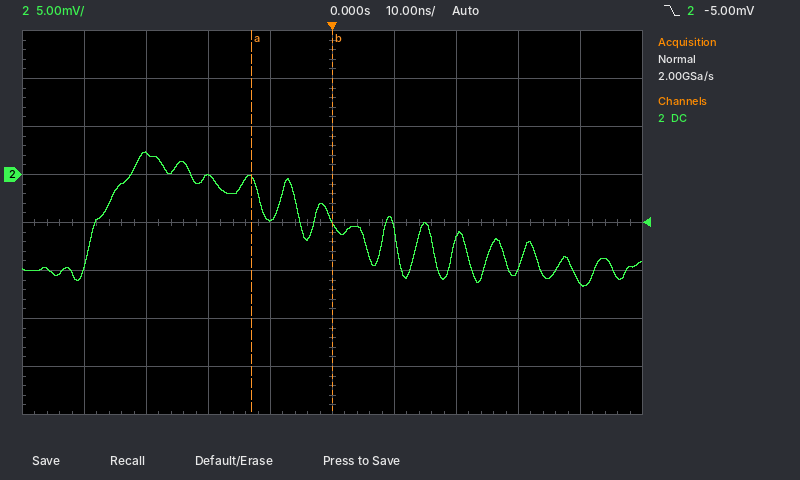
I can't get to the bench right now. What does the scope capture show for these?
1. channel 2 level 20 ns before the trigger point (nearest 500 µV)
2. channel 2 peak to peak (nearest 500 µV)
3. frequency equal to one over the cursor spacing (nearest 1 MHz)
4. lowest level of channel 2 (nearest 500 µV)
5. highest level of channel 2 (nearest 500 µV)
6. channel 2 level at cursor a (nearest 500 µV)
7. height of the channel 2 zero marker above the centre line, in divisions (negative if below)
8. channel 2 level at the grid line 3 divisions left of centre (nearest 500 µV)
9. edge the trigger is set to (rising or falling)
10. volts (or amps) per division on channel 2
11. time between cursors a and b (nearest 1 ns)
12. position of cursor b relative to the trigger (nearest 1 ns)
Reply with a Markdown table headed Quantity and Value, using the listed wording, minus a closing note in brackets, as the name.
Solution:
| Quantity | Value |
|---|---|
| channel 2 level 20 ns before the trigger point | 0.0 mV |
| channel 2 peak to peak | 14.0 mV |
| frequency equal to one over the cursor spacing | 77 MHz |
| lowest level of channel 2 | -11.5 mV |
| highest level of channel 2 | 2.5 mV |
| channel 2 level at cursor a | -500 µV |
| height of the channel 2 zero marker above the centre line, in divisions | +1.0 div |
| channel 2 level at the grid line 3 divisions left of centre | 2.0 mV |
| edge the trigger is set to | falling |
| volts (or amps) per division on channel 2 | 5 mV |
| time between cursors a and b | 13 ns |
| position of cursor b relative to the trigger | 0 ns |
